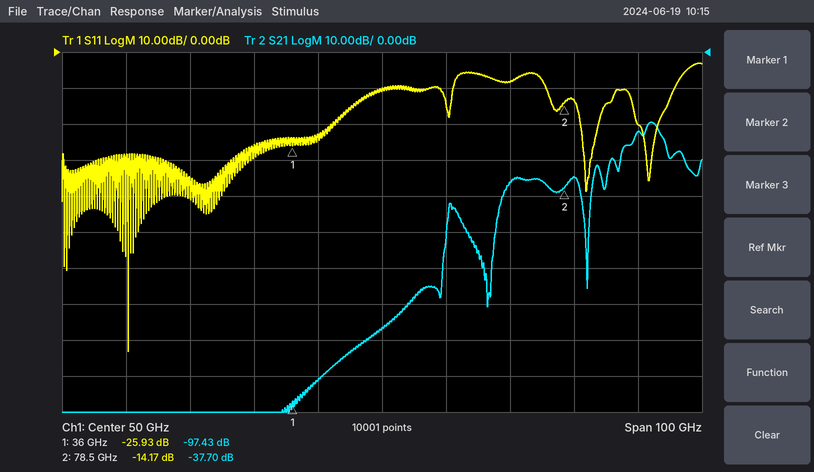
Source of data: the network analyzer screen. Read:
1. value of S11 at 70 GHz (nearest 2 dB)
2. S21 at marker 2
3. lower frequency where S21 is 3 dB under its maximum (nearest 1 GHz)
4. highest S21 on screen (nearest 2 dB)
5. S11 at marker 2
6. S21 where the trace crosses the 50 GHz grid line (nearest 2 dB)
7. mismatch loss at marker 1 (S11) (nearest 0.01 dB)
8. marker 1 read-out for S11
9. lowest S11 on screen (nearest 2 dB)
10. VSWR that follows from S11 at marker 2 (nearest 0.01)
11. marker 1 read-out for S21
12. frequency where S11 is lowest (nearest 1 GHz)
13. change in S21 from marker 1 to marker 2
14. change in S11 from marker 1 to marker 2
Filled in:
-8 dB
-37.70 dB
91 GHz
-20 dB
-14.17 dB
-76 dB
0.01 dB
-25.93 dB
-84 dB
1.49
-97.43 dB
10 GHz
59.73 dB
11.76 dB
